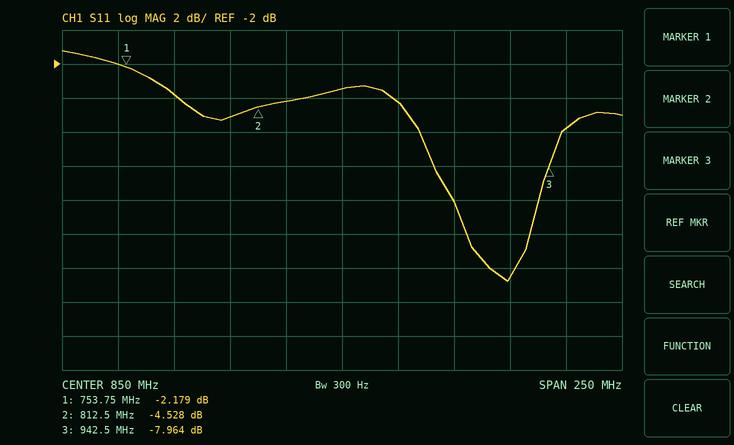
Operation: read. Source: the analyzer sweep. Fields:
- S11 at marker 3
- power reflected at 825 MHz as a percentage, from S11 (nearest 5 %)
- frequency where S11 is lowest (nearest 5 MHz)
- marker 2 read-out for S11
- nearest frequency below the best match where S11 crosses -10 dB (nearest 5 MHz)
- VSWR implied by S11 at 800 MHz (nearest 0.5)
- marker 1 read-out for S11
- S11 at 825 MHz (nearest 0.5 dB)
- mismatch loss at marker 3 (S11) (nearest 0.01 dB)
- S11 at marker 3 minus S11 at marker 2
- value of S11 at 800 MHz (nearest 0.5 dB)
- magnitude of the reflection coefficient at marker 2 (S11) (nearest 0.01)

-7.964 dB
40 %
925 MHz
-4.528 dB
900 MHz
3.5
-2.179 dB
-4.0 dB
0.76 dB
-3.436 dB
-5.0 dB
0.59
